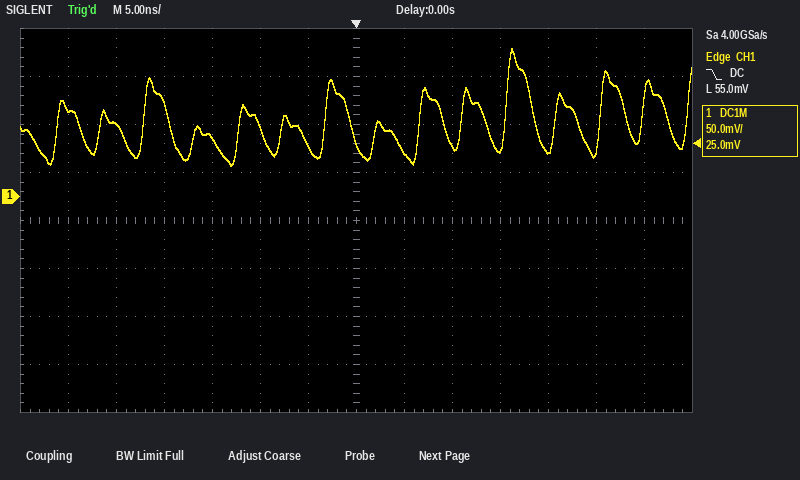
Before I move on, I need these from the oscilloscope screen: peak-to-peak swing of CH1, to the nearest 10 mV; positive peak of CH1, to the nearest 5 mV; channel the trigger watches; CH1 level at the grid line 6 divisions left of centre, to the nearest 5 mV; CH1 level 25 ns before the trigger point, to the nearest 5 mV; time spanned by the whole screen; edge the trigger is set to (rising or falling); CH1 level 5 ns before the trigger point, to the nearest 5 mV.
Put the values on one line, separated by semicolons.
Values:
120 mV; 155 mV; CH1; 90 mV; 75 mV; 70 ns; falling; 55 mV
